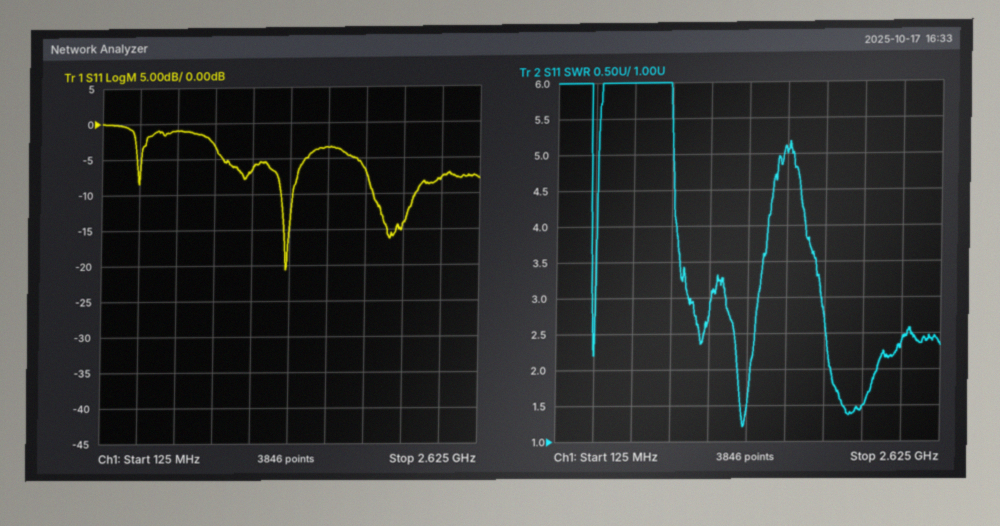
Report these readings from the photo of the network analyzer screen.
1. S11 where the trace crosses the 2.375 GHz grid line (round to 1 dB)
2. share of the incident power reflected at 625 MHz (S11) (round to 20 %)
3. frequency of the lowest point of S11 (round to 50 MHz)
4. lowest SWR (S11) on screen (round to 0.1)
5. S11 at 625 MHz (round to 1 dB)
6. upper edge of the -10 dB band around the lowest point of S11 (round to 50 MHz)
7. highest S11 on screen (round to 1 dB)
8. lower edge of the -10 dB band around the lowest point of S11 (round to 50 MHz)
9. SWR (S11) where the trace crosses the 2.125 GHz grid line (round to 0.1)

-8 dB
80 %
1.35 GHz
1.2
-1 dB
1.40 GHz
0 dB
1.30 GHz
1.5
